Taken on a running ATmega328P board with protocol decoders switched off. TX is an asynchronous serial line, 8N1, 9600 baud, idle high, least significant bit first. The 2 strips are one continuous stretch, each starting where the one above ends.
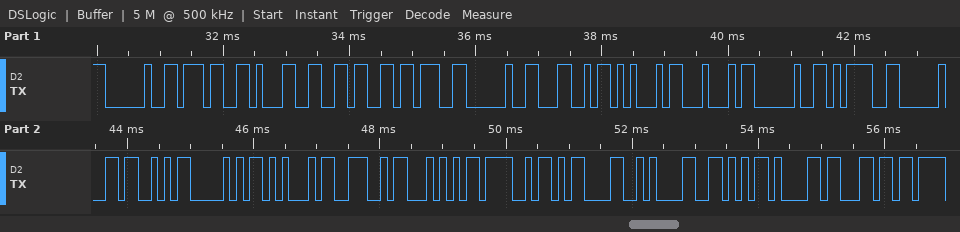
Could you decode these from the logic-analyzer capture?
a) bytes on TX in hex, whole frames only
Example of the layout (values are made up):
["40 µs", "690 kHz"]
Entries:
["20 37 31 36 3B 20 4C 45 44 20 3D 20 53 50 45 4E 54 4F 0D 0A 56 61 6C"]
